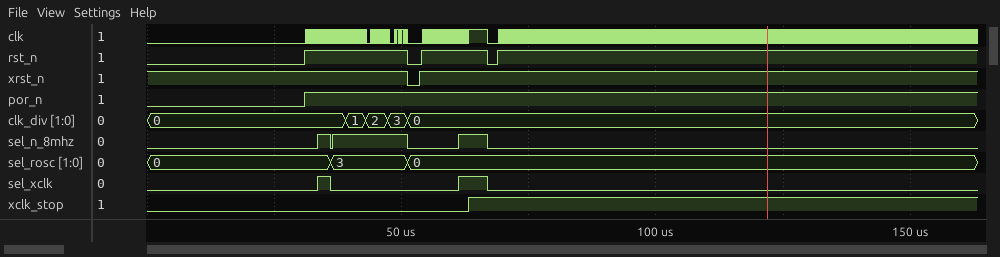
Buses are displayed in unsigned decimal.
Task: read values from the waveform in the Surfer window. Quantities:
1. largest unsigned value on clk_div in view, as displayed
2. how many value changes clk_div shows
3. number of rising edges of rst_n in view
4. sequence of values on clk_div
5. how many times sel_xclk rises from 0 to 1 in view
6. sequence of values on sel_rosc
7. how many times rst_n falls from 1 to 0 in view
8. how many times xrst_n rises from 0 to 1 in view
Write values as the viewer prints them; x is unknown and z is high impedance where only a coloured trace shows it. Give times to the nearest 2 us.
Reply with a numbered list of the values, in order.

1. 3
2. 4
3. 3
4. 0, 1, 2, 3, 0
5. 2
6. 0, 3, 0
7. 2
8. 1
